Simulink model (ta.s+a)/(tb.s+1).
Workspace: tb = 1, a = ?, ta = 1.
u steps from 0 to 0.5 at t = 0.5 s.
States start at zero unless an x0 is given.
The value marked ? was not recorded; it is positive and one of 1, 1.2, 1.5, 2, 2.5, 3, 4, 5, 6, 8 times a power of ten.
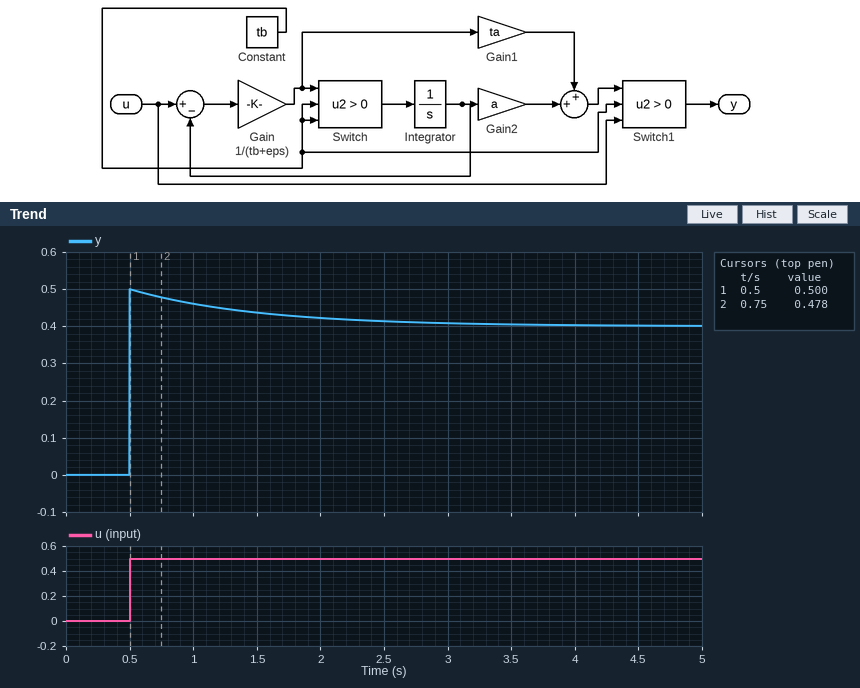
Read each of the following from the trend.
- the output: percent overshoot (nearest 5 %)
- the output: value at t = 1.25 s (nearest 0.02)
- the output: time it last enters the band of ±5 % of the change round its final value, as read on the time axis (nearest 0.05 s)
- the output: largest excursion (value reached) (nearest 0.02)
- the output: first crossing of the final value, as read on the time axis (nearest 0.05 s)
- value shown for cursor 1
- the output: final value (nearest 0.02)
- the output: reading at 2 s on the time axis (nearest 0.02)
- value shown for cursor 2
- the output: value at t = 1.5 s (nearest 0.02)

25 %
0.44
2.10 s
0.50
0.50 s
0.500
0.40
0.42
0.478
0.44
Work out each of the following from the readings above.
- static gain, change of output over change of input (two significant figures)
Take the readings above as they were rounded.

0.80
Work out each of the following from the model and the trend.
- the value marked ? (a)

0.8
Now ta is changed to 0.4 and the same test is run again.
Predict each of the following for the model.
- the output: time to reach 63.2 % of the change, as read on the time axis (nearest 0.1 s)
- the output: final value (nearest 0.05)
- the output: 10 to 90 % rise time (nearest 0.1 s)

0.8 s
0.40
1.6 s
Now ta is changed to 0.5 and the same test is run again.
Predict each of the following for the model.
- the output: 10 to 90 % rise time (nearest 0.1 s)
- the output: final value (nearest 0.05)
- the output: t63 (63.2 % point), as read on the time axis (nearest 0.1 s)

1.3 s
0.40
0.5 s
